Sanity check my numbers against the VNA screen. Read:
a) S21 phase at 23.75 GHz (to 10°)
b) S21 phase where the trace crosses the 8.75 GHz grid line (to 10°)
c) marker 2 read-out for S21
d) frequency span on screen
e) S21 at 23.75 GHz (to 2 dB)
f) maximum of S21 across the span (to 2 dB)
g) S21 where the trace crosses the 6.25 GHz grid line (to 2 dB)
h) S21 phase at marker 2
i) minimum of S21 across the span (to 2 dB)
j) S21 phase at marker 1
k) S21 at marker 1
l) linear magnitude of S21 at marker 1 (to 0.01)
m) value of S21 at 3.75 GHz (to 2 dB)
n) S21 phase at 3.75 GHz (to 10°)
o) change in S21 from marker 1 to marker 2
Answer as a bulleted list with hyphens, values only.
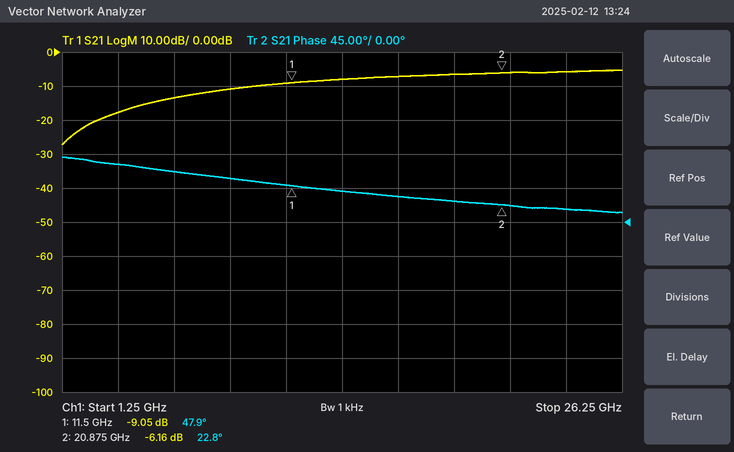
- 20°
- 60°
- -6.16 dB
- 25 GHz
- -6 dB
- -6 dB
- -14 dB
- 22.8°
- -28 dB
- 47.9°
- -9.05 dB
- 0.35
- -18 dB
- 80°
- 2.89 dB
